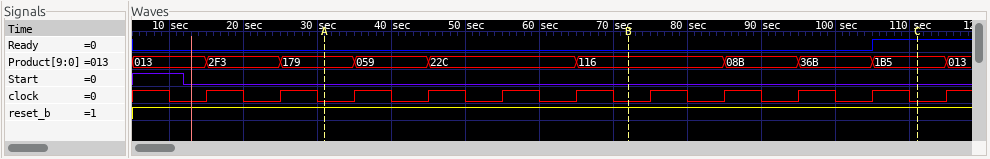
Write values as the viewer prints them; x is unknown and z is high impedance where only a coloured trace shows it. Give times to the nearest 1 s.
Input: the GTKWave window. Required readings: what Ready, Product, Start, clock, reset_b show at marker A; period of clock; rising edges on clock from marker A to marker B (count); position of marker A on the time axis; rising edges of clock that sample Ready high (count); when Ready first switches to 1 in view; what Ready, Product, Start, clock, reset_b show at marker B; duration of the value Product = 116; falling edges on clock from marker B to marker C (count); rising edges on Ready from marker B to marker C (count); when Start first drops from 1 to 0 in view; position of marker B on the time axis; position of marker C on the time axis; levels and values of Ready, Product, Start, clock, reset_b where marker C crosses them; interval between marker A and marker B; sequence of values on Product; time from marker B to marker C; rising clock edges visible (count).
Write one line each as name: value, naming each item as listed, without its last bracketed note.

what Ready, Product, Start, clock, reset_b show at marker A: Ready=0, Product=179, Start=0, clock=0, reset_b=1
period of clock: 10 s
rising edges on clock from marker A to marker B: 4
position of marker A on the time axis: 31 s
rising edges of clock that sample Ready high: 1
when Ready first switches to 1 in view: 105 s
what Ready, Product, Start, clock, reset_b show at marker B: Ready=0, Product=116, Start=0, clock=0, reset_b=1
duration of the value Product = 116: 20 s
falling edges on clock from marker B to marker C: 4
rising edges on Ready from marker B to marker C: 1
when Start first drops from 1 to 0 in view: 12 s
position of marker B on the time axis: 72 s
position of marker C on the time axis: 111 s
levels and values of Ready, Product, Start, clock, reset_b where marker C crosses them: Ready=1, Product=1B5, Start=0, clock=0, reset_b=1
interval between marker A and marker B: 41 s
sequence of values on Product: 013, 2F3, 179, 059, 22C, 116, 08B, 36B, 1B5, 013
time from marker B to marker C: 39 s
rising clock edges visible: 11
